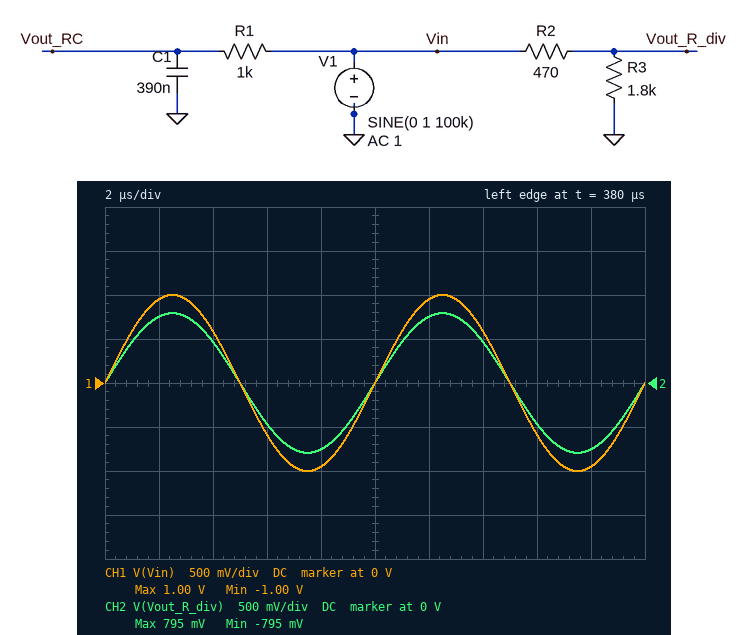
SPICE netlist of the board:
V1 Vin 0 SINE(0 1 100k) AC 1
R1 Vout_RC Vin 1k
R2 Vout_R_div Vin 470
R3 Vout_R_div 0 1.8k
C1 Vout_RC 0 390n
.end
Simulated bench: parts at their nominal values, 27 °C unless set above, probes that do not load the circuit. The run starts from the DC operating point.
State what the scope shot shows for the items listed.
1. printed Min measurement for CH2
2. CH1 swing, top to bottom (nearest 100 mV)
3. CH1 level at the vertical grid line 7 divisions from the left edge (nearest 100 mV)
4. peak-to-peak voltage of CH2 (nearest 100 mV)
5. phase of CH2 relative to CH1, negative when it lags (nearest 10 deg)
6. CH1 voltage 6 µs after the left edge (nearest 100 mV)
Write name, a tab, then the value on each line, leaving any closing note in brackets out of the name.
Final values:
printed Min measurement for CH2	-795 mV
CH1 swing, top to bottom	2.0 V
CH1 level at the vertical grid line 7 divisions from the left edge	600 mV
peak-to-peak voltage of CH2	1.6 V
phase of CH2 relative to CH1, negative when it lags	0 deg
CH1 voltage 6 µs after the left edge	-600 mV
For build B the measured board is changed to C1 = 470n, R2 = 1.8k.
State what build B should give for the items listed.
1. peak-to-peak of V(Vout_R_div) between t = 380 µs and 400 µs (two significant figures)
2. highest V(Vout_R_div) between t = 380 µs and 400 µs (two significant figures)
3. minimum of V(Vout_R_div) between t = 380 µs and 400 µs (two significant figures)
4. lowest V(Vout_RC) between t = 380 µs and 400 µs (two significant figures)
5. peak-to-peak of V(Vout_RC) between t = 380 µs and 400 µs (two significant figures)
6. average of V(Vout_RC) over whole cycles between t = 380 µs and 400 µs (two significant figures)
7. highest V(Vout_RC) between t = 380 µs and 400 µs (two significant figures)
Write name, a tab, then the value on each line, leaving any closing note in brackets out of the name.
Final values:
peak-to-peak of V(Vout_R_div) between t = 380 µs and 400 µs	1.0 V
highest V(Vout_R_div) between t = 380 µs and 400 µs	500 mV
minimum of V(Vout_R_div) between t = 380 µs and 400 µs	-500 mV
lowest V(Vout_RC) between t = 380 µs and 400 µs	-1.9 mV
peak-to-peak of V(Vout_RC) between t = 380 µs and 400 µs	6.8 mV
average of V(Vout_RC) over whole cycles between t = 380 µs and 400 µs	1.5 mV
highest V(Vout_RC) between t = 380 µs and 400 µs	4.9 mV
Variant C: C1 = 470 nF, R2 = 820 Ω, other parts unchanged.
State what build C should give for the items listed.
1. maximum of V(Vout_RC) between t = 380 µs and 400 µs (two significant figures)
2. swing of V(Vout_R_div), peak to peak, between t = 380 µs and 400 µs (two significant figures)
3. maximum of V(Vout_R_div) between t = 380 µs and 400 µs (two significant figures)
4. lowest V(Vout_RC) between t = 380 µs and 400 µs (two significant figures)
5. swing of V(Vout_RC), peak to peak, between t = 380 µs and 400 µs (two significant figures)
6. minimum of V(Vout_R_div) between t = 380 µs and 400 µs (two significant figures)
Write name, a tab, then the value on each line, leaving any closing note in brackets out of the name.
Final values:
maximum of V(Vout_RC) between t = 380 µs and 400 µs	4.9 mV
swing of V(Vout_R_div), peak to peak, between t = 380 µs and 400 µs	1.4 V
maximum of V(Vout_R_div) between t = 380 µs and 400 µs	690 mV
lowest V(Vout_RC) between t = 380 µs and 400 µs	-1.9 mV
swing of V(Vout_RC), peak to peak, between t = 380 µs and 400 µs	6.8 mV
minimum of V(Vout_R_div) between t = 380 µs and 400 µs	-690 mV
